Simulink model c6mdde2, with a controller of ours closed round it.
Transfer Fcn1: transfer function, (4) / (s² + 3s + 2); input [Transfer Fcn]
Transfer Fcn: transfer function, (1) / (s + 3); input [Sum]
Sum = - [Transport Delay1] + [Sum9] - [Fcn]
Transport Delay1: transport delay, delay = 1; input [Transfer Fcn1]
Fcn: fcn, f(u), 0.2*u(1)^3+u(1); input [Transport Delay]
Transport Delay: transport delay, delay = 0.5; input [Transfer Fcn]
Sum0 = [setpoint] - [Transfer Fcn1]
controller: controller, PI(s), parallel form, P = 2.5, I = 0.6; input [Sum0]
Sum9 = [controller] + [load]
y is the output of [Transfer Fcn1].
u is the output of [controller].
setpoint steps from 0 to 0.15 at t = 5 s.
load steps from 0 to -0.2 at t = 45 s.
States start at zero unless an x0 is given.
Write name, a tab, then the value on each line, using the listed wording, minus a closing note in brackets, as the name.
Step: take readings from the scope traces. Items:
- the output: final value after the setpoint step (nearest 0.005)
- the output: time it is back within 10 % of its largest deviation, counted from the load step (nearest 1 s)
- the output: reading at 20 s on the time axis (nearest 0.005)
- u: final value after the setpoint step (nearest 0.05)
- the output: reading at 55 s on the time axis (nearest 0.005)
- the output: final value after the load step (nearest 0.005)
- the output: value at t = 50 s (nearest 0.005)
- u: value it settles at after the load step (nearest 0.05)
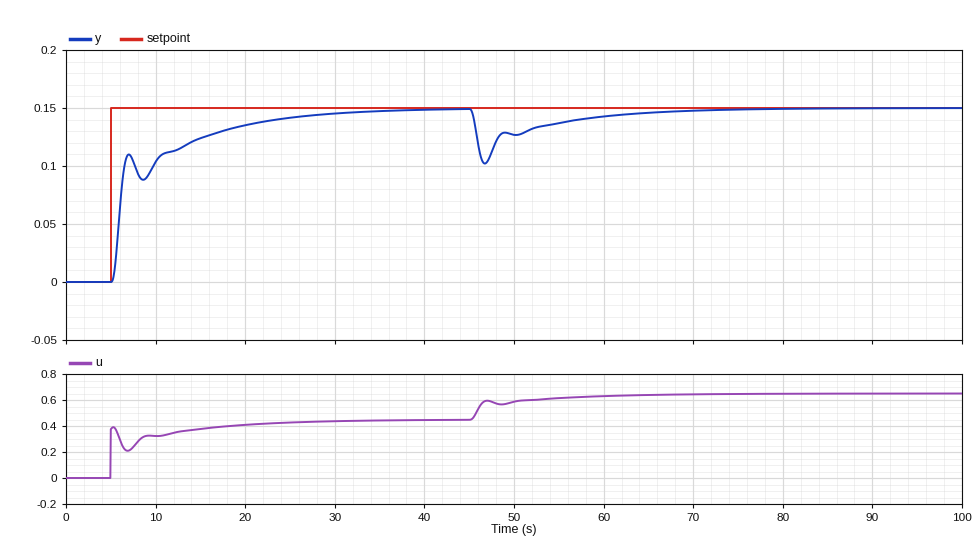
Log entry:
the output: final value after the setpoint step	0.150
the output: time it is back within 10 % of its largest deviation, counted from the load step	19 s
the output: reading at 20 s on the time axis	0.135
u: final value after the setpoint step	0.45
the output: reading at 55 s on the time axis	0.135
the output: final value after the load step	0.150
the output: value at t = 50 s	0.125
u: value it settles at after the load step	0.65
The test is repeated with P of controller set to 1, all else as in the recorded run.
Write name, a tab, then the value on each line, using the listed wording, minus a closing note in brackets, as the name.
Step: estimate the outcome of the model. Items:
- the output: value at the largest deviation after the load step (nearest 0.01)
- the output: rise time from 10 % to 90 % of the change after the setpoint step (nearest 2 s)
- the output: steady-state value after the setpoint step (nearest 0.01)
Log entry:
the output: value at the largest deviation after the load step	0.09
the output: rise time from 10 % to 90 % of the change after the setpoint step	12 s
the output: steady-state value after the setpoint step	0.15
